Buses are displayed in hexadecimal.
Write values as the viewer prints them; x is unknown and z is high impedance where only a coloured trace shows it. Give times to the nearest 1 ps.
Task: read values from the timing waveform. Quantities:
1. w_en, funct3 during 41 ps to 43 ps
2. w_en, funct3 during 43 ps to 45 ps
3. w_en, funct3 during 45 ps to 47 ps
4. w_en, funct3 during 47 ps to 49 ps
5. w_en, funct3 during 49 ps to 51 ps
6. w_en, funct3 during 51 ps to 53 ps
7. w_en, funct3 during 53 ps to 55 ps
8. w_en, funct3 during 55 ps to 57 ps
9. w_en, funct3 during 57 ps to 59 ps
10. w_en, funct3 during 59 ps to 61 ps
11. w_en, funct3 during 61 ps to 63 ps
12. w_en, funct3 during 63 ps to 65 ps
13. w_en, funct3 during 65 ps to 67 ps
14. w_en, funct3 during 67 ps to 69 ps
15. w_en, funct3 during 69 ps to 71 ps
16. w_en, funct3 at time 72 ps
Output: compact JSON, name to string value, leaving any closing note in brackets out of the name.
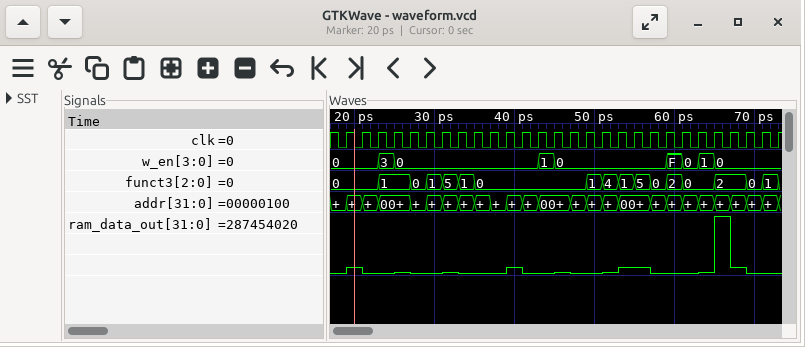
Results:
{"w_en, funct3 during 41 ps to 43 ps": "w_en=0, funct3=0", "w_en, funct3 during 43 ps to 45 ps": "w_en=1, funct3=0", "w_en, funct3 during 45 ps to 47 ps": "w_en=0, funct3=0", "w_en, funct3 during 47 ps to 49 ps": "w_en=0, funct3=0", "w_en, funct3 during 49 ps to 51 ps": "w_en=0, funct3=1", "w_en, funct3 during 51 ps to 53 ps": "w_en=0, funct3=4", "w_en, funct3 during 53 ps to 55 ps": "w_en=0, funct3=1", "w_en, funct3 during 55 ps to 57 ps": "w_en=0, funct3=5", "w_en, funct3 during 57 ps to 59 ps": "w_en=0, funct3=0", "w_en, funct3 during 59 ps to 61 ps": "w_en=F, funct3=2", "w_en, funct3 during 61 ps to 63 ps": "w_en=0, funct3=0", "w_en, funct3 during 63 ps to 65 ps": "w_en=1, funct3=0", "w_en, funct3 during 65 ps to 67 ps": "w_en=0, funct3=2", "w_en, funct3 during 67 ps to 69 ps": "w_en=0, funct3=2", "w_en, funct3 during 69 ps to 71 ps": "w_en=0, funct3=0", "w_en, funct3 at time 72 ps": "w_en=0, funct3=1"}
